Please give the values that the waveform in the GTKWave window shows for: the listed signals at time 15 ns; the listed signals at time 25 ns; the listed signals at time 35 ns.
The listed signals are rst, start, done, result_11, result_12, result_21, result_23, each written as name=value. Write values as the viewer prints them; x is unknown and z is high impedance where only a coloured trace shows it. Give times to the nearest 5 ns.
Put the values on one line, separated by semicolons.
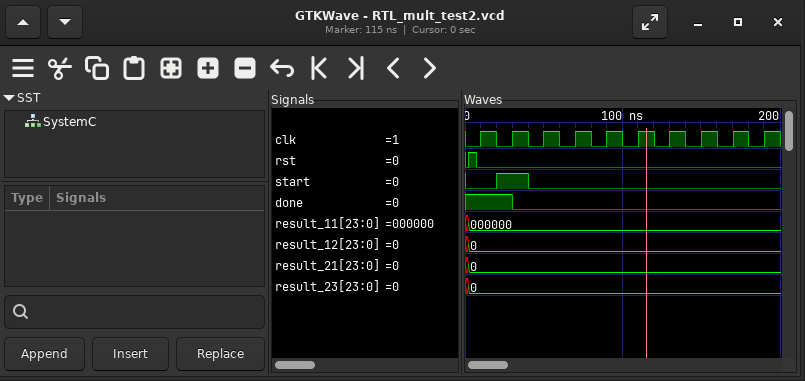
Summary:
rst=0, start=0, done=1, result_11=000000, result_12=0, result_21=0, result_23=0; rst=0, start=1, done=1, result_11=000000, result_12=0, result_21=0, result_23=0; rst=0, start=1, done=0, result_11=000000, result_12=0, result_21=0, result_23=0
